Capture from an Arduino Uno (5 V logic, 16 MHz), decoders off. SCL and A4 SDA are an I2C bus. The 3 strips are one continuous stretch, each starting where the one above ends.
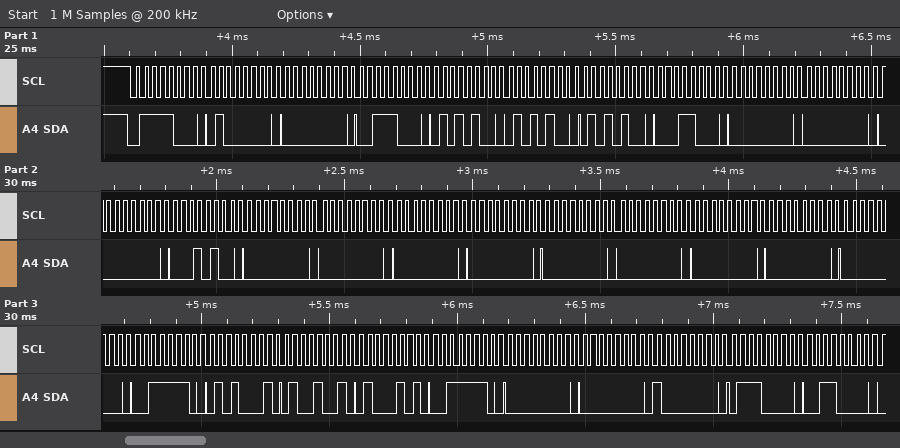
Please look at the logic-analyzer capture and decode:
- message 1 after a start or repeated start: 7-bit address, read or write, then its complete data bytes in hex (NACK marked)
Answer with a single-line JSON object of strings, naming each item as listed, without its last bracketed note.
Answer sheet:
{"message 1 after a start or repeated start: 7-bit address, read or write, then its complete data bytes in hex": "0x3C write: 40 00 38 54 54 54 18 00 00 00 14 00 00 00 00 00 00 00 00 00 3E 51 49 45 3E 00 00 80 70 30"}
